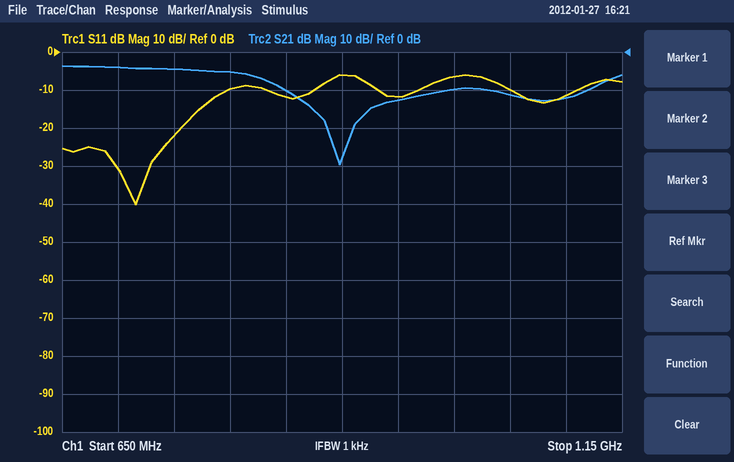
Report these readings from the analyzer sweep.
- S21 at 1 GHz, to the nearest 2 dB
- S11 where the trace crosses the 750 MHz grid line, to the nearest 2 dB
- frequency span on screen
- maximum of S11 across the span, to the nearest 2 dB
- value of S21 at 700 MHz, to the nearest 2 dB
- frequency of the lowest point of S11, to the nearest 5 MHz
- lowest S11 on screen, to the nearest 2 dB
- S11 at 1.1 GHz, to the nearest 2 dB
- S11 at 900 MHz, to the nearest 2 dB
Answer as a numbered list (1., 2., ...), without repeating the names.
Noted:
1. -10 dB
2. -22 dB
3. 500 MHz
4. -6 dB
5. -4 dB
6. 715 MHz
7. -40 dB
8. -12 dB
9. -6 dB
